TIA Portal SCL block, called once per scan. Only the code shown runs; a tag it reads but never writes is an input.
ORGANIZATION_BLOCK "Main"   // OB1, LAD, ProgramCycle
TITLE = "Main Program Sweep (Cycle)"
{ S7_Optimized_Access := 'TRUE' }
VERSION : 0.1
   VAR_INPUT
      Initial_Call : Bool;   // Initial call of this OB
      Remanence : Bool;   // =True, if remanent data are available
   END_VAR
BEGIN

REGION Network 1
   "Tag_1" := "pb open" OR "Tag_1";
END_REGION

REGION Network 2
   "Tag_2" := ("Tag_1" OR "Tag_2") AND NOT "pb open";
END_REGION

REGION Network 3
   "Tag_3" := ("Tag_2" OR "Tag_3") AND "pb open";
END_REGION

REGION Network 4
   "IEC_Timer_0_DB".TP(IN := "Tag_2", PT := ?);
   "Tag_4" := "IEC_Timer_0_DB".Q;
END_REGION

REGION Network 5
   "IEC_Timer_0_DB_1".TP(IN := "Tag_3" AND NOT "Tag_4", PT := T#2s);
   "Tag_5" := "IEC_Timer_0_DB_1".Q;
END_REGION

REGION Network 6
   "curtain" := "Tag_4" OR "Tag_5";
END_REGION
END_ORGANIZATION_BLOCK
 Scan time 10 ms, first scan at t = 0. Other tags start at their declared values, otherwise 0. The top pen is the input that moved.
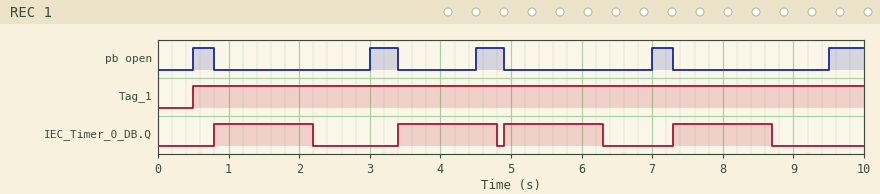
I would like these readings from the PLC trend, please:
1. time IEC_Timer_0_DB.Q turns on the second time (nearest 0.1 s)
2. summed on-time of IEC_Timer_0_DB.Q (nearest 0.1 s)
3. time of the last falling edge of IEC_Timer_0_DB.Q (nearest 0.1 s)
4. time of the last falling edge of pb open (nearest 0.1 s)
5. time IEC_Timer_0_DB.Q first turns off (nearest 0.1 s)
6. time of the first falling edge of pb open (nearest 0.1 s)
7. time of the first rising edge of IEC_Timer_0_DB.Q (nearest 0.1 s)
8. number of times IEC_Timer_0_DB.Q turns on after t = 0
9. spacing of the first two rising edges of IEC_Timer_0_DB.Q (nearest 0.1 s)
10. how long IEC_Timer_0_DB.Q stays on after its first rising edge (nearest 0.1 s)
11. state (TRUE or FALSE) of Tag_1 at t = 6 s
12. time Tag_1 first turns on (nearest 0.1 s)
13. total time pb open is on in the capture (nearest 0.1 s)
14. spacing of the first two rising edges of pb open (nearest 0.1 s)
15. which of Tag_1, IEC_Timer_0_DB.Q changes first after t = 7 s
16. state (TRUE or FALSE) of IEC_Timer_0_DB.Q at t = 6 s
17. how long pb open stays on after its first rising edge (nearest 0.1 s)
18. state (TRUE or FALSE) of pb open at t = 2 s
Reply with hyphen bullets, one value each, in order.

- 3.4 s
- 5.6 s
- 8.7 s
- 7.3 s
- 2.2 s
- 0.8 s
- 0.8 s
- 4
- 2.6 s
- 1.4 s
- TRUE
- 0.5 s
- 1.9 s
- 2.5 s
- IEC_Timer_0_DB.Q
- TRUE
- 0.3 s
- FALSE
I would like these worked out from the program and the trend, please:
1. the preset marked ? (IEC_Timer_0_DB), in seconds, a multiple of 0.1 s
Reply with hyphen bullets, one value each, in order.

- 1.4 s
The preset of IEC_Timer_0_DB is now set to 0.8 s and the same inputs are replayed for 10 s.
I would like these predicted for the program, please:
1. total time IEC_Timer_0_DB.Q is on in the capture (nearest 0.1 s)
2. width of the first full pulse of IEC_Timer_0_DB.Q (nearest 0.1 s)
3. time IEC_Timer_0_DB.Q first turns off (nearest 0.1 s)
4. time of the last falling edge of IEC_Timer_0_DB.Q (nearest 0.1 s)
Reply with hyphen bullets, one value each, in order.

- 3.2 s
- 0.8 s
- 1.6 s
- 8.1 s
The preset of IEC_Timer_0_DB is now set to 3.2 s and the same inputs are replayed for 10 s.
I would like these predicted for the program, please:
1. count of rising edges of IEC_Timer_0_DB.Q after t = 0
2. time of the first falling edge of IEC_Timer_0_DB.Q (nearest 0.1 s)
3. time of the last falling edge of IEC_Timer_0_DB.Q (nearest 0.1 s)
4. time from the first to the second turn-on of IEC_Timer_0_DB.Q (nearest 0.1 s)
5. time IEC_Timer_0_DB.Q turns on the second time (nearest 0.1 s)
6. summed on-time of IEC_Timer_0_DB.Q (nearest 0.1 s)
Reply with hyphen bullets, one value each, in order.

- 2
- 4.0 s
- 8.1 s
- 4.1 s
- 4.9 s
- 6.4 s
